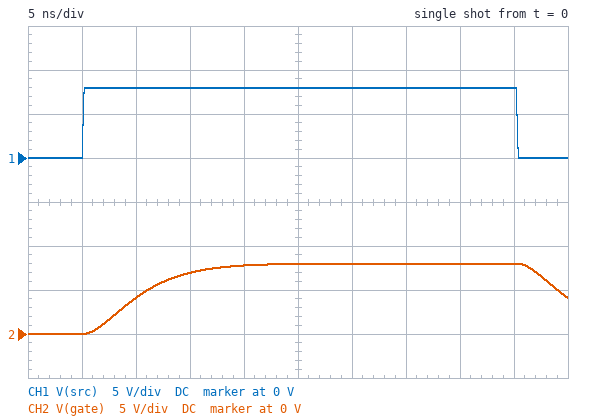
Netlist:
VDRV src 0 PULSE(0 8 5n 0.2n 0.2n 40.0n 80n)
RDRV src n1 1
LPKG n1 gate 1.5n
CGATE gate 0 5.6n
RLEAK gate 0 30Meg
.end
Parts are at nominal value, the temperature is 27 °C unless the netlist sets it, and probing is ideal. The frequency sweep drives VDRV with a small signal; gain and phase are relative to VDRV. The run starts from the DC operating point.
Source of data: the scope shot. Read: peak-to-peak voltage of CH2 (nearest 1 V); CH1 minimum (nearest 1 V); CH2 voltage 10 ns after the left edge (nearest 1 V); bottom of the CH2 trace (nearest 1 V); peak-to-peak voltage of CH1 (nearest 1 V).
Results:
8 V
0 V
4 V
0 V
8 V
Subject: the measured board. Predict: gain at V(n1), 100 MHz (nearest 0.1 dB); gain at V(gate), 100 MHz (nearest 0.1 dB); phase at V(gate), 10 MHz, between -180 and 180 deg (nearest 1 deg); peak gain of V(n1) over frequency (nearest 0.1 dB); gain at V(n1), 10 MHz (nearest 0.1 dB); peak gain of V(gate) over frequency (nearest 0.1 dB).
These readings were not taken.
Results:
-5.2 dB
-12.5 dB
-20 deg
0 dB
-0.5 dB
0 dB
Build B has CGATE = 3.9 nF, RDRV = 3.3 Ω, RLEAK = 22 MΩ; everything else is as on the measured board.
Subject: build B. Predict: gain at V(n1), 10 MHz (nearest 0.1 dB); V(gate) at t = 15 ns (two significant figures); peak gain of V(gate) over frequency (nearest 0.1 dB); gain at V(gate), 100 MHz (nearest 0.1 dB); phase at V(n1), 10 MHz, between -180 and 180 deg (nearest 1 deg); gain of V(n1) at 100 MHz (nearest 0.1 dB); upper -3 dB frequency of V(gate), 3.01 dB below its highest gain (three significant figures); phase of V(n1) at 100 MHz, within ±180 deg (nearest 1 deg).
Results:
-2.3 dB
4.3 V
0 dB
-18.3 dB
-40 deg
-15.9 dB
12.8 MHz
81 deg
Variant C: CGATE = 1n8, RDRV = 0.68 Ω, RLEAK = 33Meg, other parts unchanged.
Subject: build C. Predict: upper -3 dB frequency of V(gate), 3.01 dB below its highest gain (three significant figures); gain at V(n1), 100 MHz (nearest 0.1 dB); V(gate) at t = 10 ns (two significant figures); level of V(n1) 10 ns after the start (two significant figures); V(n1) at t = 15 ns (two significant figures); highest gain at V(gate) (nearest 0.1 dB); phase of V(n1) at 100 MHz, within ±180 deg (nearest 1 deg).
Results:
115 MHz
-21.4 dB
10 V
7.2 V
8.4 V
3.2 dB
85 deg
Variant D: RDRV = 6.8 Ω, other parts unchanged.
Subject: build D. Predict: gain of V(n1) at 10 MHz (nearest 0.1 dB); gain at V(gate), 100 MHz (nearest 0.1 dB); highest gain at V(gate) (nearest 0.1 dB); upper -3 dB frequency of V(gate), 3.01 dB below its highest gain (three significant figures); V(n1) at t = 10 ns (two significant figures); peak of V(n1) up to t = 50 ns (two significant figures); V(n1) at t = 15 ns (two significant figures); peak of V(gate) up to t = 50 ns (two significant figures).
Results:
-8.5 dB
-27.6 dB
0 dB
4.20 MHz
890 mV
5.3 V
1.8 V
5.2 V
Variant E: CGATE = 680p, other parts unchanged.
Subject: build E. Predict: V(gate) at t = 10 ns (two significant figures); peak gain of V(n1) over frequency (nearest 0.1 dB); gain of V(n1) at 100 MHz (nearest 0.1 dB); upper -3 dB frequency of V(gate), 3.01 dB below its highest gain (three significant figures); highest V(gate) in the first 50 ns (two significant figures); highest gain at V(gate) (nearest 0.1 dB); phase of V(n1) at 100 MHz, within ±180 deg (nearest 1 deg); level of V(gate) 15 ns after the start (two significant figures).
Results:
8.8 V
0 dB
-1.8 dB
187 MHz
11 V
4.0 dB
-36 deg
8.3 V
